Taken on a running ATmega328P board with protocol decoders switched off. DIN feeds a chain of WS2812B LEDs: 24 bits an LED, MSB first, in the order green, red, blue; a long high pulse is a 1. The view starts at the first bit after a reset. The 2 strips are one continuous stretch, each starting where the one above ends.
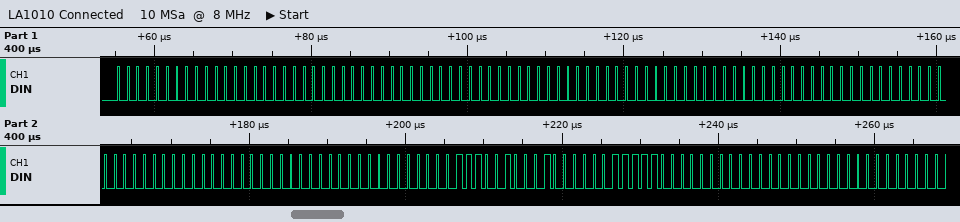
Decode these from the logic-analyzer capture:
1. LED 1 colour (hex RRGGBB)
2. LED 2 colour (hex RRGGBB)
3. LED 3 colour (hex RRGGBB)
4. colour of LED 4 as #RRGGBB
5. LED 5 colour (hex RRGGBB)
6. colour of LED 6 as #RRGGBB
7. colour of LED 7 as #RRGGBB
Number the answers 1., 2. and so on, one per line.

1. #000000
2. #000000
3. #000000
4. #000000
5. #000000
6. #20727C
7. #000000
